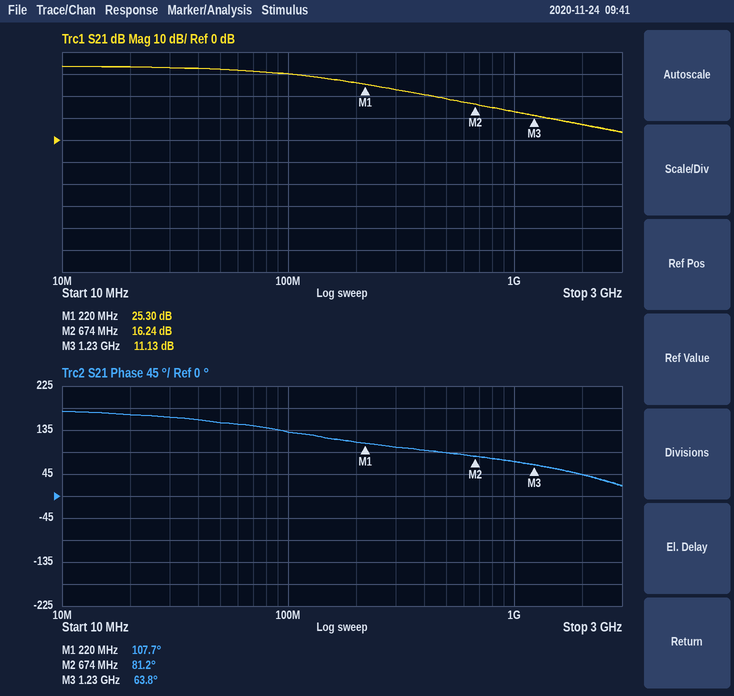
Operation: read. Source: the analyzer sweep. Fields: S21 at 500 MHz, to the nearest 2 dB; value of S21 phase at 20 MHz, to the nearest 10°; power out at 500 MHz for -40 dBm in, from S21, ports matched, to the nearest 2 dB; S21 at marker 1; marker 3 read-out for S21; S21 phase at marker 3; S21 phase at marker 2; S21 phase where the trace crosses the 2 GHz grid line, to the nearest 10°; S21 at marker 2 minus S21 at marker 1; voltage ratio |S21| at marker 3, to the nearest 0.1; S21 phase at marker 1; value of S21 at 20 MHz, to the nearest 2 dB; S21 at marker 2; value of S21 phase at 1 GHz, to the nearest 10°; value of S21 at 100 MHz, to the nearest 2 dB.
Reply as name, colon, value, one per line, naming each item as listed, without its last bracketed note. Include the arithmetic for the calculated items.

S21 at 500 MHz, to the nearest 2 dB: 18 dB
value of S21 phase at 20 MHz, to the nearest 10°: 170°
power out at 500 MHz for -40 dBm in, from S21, ports matched, to the nearest 2 dB: -40 dBm + (18 dB) = -22 dBm
S21 at marker 1: 25.30 dB
marker 3 read-out for S21: 11.13 dB
S21 phase at marker 3: 63.8°
S21 phase at marker 2: 81.2°
S21 phase where the trace crosses the 2 GHz grid line, to the nearest 10°: 40°
S21 at marker 2 minus S21 at marker 1: 16.24 − (25.3) = -9.06 dB
voltage ratio |S21| at marker 3, to the nearest 0.1: 10^(11.13/20) ≈ 3.6
S21 phase at marker 1: 107.7°
value of S21 at 20 MHz, to the nearest 2 dB: 34 dB
S21 at marker 2: 16.24 dB
value of S21 phase at 1 GHz, to the nearest 10°: 70°
value of S21 at 100 MHz, to the nearest 2 dB: 30 dB
